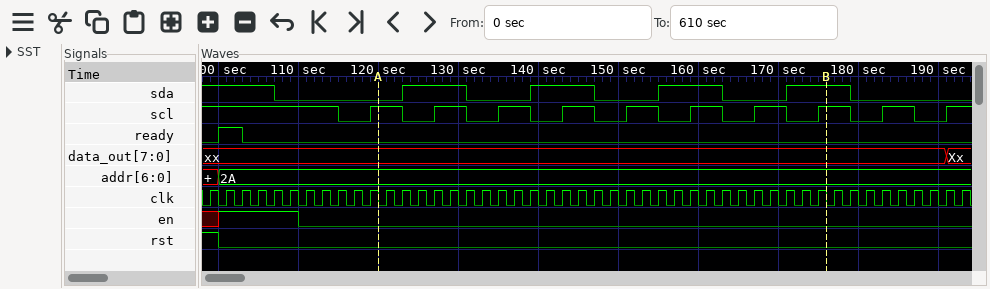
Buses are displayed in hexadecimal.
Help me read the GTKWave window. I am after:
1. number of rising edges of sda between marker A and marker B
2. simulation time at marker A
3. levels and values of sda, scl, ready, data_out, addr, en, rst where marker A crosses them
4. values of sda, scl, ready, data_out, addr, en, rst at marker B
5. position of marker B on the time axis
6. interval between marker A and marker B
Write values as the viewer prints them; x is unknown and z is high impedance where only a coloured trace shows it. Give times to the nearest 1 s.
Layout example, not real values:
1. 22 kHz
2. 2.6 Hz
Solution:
1. 4
2. 120 s
3. sda=0, scl=1, ready=0, data_out=xx, addr=2A, en=0, rst=0
4. sda=1, scl=1, ready=0, data_out=xx, addr=2A, en=0, rst=0
5. 176 s
6. 56 s
